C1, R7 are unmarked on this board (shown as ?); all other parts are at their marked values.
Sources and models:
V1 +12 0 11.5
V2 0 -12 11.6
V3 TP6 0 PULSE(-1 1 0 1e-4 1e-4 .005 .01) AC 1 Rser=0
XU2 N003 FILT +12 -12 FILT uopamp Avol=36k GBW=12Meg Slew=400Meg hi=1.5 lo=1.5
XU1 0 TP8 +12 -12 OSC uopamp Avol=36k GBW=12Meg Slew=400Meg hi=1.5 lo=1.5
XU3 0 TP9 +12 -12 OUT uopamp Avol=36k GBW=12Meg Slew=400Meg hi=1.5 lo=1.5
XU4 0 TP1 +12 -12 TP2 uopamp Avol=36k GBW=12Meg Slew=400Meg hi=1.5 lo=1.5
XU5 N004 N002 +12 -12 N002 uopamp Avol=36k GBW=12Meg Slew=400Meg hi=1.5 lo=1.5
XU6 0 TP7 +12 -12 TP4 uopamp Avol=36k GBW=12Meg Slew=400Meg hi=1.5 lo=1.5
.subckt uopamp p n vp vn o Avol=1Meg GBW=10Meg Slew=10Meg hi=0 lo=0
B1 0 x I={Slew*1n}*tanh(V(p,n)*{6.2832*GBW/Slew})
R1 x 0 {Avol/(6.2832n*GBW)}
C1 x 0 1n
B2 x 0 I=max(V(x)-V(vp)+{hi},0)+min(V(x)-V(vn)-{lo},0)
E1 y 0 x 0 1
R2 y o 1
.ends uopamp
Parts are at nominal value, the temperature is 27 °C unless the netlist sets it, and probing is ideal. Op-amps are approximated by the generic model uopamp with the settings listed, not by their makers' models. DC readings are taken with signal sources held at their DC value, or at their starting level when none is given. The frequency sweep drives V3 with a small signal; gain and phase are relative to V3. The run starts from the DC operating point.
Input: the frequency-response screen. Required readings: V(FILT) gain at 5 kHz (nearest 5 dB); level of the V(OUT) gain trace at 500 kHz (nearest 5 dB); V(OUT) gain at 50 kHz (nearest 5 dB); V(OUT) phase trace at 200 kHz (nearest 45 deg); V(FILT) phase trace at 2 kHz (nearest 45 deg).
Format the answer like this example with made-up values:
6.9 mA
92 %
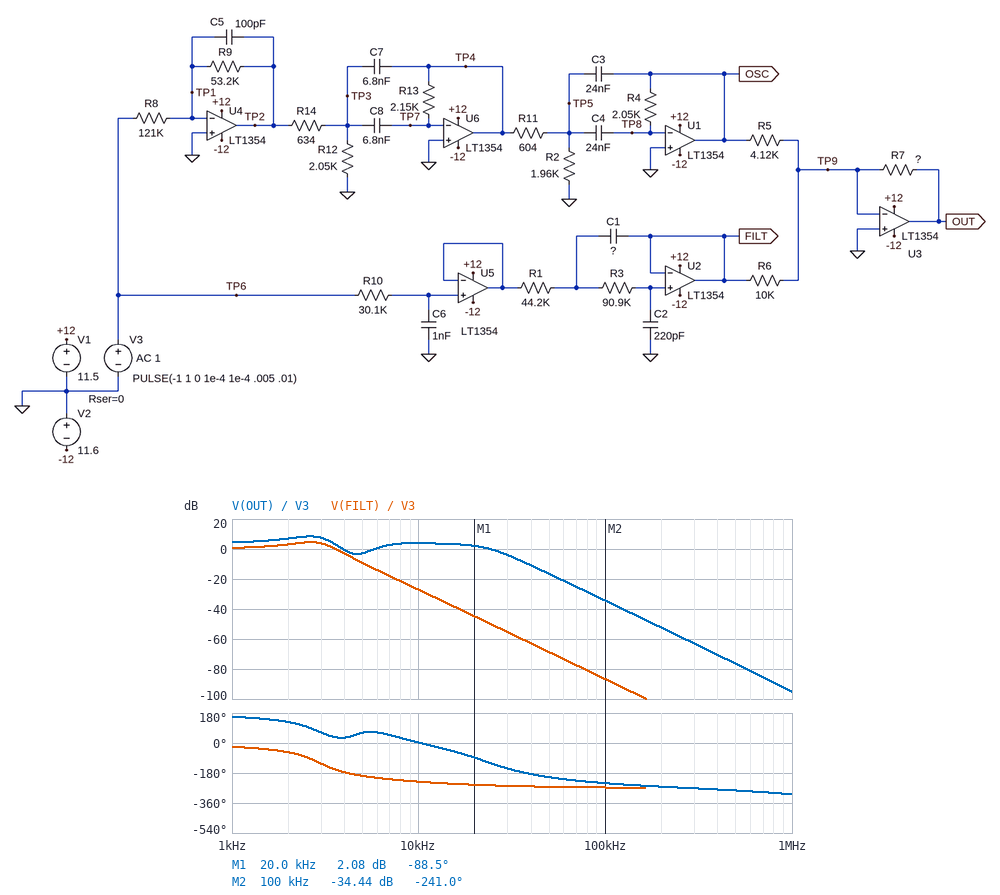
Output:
-10 dB
-75 dB
-15 dB
-270 deg
-45 deg
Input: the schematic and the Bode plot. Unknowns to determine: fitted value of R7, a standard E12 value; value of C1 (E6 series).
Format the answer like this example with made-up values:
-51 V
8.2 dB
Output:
15 kΩ
3.3 nF
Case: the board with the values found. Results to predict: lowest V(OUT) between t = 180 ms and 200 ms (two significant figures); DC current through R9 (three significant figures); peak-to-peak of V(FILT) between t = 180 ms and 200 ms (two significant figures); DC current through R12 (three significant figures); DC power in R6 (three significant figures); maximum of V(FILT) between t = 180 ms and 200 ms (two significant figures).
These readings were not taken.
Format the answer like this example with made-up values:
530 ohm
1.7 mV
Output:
-2.4 V
8.26 µA
3.2 V
164 µA
100 µW
1.6 V
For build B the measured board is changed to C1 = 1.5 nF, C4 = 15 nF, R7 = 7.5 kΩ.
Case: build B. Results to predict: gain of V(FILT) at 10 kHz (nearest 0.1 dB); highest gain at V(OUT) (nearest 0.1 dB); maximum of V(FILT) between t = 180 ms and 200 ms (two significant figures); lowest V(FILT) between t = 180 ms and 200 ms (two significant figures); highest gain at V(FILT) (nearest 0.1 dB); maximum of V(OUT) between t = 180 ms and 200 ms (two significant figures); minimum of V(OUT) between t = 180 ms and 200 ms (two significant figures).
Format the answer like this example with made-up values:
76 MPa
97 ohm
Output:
-19.9 dB
-0.8 dB
1.2 V
-1.2 V
1.1 dB
920 mV
-920 mV
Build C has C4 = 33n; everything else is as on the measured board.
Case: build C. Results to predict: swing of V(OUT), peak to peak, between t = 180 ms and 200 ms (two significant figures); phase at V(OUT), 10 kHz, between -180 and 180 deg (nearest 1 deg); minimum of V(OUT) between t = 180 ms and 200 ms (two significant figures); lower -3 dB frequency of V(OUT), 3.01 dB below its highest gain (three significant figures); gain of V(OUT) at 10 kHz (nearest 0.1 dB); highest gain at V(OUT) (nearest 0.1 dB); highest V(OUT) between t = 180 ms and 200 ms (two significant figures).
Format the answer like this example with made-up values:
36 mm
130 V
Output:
4.7 V
-8 deg
-2.3 V
1.51 kHz
3.7 dB
8.6 dB
2.3 V
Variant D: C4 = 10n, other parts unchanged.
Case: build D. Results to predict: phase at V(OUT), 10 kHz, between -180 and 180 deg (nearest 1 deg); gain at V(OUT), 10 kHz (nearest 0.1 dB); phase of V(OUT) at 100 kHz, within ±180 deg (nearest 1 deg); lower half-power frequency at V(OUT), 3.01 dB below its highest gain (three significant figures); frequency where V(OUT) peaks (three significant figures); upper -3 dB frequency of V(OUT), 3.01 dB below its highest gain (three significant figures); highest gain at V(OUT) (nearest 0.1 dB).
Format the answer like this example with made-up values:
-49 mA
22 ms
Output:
47 deg
1.2 dB
122 deg
1.43 kHz
2.64 kHz
3.34 kHz
8.2 dB
